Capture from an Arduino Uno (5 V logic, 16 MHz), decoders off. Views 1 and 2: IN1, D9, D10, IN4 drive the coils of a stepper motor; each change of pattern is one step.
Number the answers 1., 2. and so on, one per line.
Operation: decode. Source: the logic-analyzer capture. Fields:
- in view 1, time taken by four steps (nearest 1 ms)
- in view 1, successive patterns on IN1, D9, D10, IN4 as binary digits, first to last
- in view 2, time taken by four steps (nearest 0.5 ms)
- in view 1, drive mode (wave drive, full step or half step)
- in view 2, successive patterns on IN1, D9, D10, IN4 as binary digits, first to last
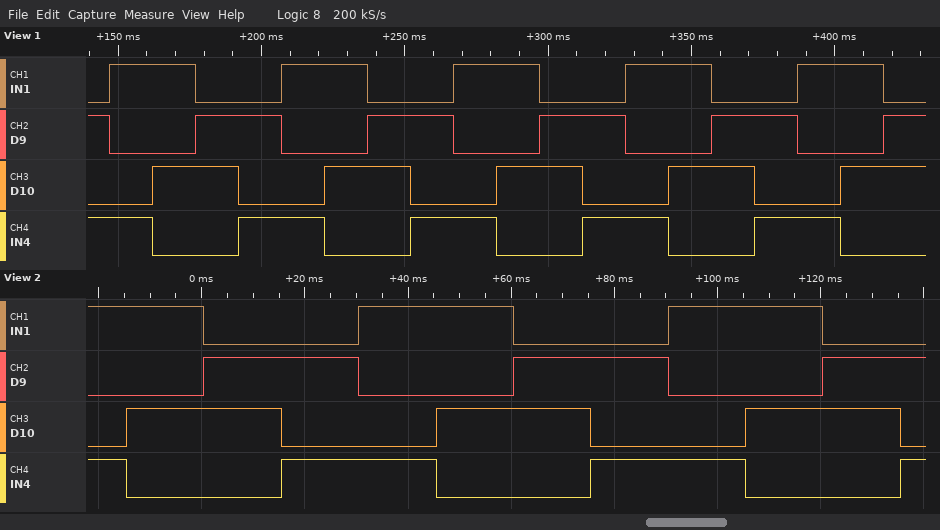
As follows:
1. 60 ms
2. 0101 1001 1010 0110 0101 1001 1010 0110 0101 1001 1010 0110 0101 1001 1010 0110 0101 1001 1010 0110
3. 60.0 ms
4. full step
5. 1001 1010 0110 0101 1001 1010 0110 0101 1001 1010 0110 0101
